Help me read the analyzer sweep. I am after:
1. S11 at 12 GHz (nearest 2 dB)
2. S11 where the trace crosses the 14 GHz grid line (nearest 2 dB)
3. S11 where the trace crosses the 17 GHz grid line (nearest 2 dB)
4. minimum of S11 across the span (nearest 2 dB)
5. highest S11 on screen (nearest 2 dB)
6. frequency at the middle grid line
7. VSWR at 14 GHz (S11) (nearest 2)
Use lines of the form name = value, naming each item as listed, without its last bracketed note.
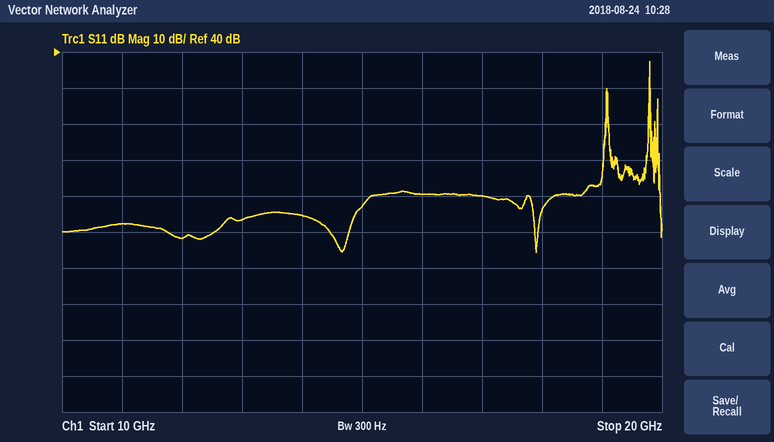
S11 at 12 GHz = -12 dB
S11 where the trace crosses the 14 GHz grid line = -6 dB
S11 where the trace crosses the 17 GHz grid line = 0 dB
minimum of S11 across the span = -16 dB
highest S11 on screen = 38 dB
frequency at the middle grid line = 15 GHz
VSWR at 14 GHz (S11) = 4
